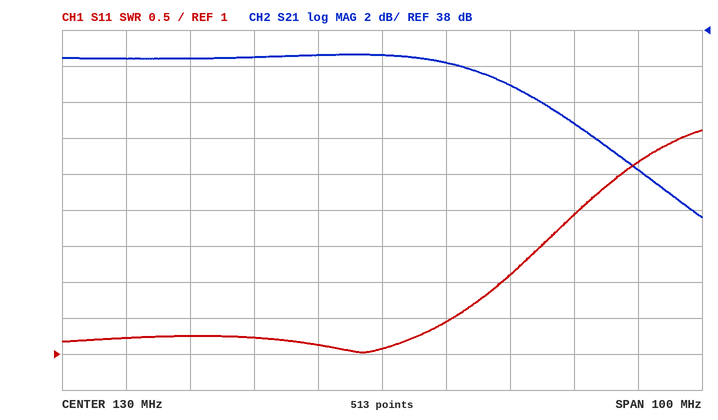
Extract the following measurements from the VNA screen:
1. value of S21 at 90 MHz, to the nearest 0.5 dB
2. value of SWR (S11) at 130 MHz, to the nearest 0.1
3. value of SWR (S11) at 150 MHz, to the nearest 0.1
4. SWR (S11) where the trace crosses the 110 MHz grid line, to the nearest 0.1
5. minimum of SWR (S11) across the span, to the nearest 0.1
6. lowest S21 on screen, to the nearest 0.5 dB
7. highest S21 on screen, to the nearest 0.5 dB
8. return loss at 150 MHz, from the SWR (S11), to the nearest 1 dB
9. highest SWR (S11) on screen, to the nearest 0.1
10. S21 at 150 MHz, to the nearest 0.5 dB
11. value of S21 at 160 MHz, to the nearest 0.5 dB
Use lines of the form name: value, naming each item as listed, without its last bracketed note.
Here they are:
value of S21 at 90 MHz, to the nearest 0.5 dB: 36.5 dB
value of SWR (S11) at 130 MHz, to the nearest 0.1: 1.1
value of SWR (S11) at 150 MHz, to the nearest 0.1: 2.1
SWR (S11) where the trace crosses the 110 MHz grid line, to the nearest 0.1: 1.2
minimum of SWR (S11) across the span, to the nearest 0.1: 1.0
lowest S21 on screen, to the nearest 0.5 dB: 27.5 dB
highest S21 on screen, to the nearest 0.5 dB: 36.5 dB
return loss at 150 MHz, from the SWR (S11), to the nearest 1 dB: 9 dB
highest SWR (S11) on screen, to the nearest 0.1: 4.1
S21 at 150 MHz, to the nearest 0.5 dB: 35.0 dB
value of S21 at 160 MHz, to the nearest 0.5 dB: 33.0 dB
